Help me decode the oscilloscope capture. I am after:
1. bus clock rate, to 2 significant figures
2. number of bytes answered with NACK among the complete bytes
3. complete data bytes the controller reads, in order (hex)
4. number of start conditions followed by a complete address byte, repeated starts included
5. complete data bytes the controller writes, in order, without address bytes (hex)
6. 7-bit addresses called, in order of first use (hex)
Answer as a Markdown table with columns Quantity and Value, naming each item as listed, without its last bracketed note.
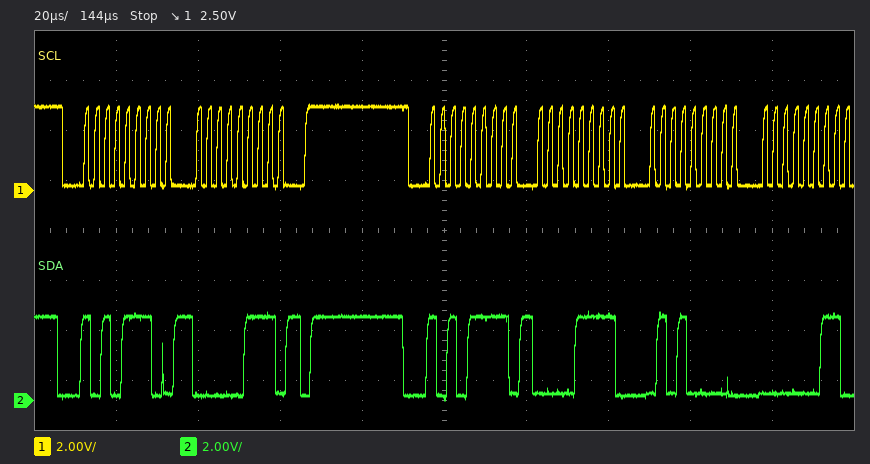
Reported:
| Quantity | Value |
|---|---|
| bus clock rate, to 2 significant figures | 400 kHz |
| number of bytes answered with NACK among the complete bytes | 0 |
| complete data bytes the controller reads, in order | 0F 50 03 |
| number of start conditions followed by a complete address byte, repeated starts included | 2 |
| complete data bytes the controller writes, in order, without address bytes | 07 |
| 7-bit addresses called, in order of first use | 0x57 |
